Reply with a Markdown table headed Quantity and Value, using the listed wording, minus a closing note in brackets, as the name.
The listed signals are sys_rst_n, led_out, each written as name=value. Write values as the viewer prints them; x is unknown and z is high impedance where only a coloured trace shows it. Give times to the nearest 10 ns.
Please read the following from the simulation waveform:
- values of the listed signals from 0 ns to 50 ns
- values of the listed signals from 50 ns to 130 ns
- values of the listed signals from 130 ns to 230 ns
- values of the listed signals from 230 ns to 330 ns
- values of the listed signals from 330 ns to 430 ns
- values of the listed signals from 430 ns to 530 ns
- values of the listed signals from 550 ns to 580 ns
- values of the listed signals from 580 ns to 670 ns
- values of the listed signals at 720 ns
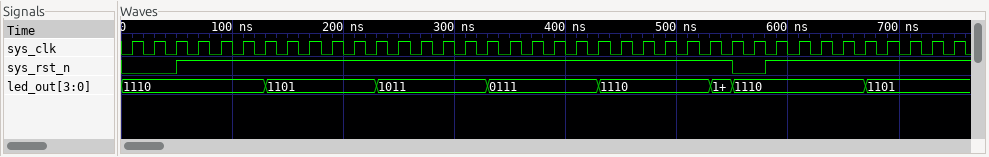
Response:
| Quantity | Value |
|---|---|
| values of the listed signals from 0 ns to 50 ns | sys_rst_n=0, led_out=1110 |
| values of the listed signals from 50 ns to 130 ns | sys_rst_n=1, led_out=1110 |
| values of the listed signals from 130 ns to 230 ns | sys_rst_n=1, led_out=1101 |
| values of the listed signals from 230 ns to 330 ns | sys_rst_n=1, led_out=1011 |
| values of the listed signals from 330 ns to 430 ns | sys_rst_n=1, led_out=0111 |
| values of the listed signals from 430 ns to 530 ns | sys_rst_n=1, led_out=1110 |
| values of the listed signals from 550 ns to 580 ns | sys_rst_n=0, led_out=1110 |
| values of the listed signals from 580 ns to 670 ns | sys_rst_n=1, led_out=1110 |
| values of the listed signals at 720 ns | sys_rst_n=1, led_out=1101 |
